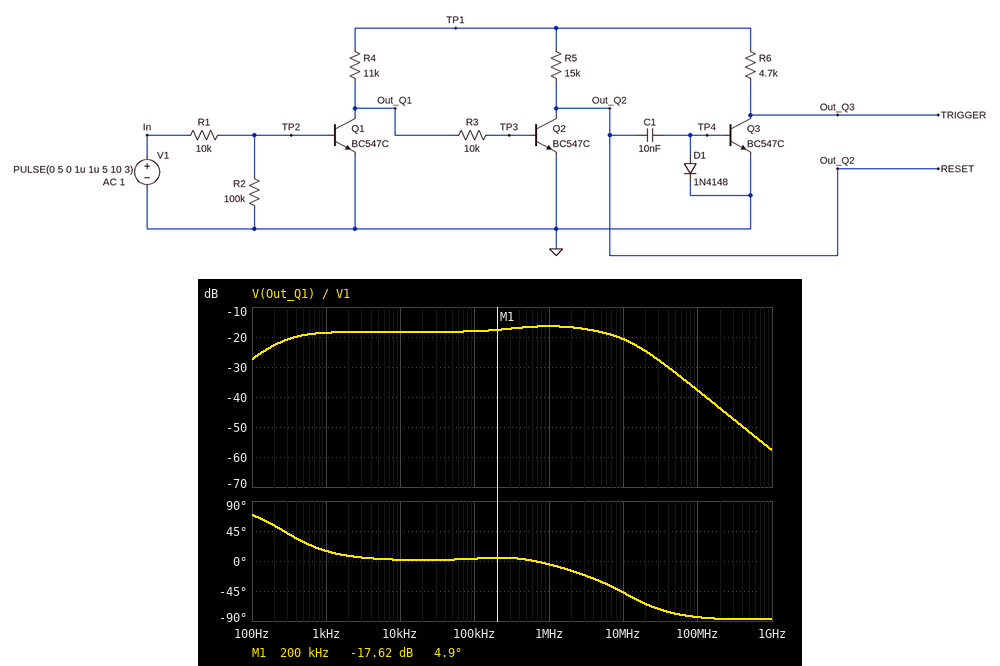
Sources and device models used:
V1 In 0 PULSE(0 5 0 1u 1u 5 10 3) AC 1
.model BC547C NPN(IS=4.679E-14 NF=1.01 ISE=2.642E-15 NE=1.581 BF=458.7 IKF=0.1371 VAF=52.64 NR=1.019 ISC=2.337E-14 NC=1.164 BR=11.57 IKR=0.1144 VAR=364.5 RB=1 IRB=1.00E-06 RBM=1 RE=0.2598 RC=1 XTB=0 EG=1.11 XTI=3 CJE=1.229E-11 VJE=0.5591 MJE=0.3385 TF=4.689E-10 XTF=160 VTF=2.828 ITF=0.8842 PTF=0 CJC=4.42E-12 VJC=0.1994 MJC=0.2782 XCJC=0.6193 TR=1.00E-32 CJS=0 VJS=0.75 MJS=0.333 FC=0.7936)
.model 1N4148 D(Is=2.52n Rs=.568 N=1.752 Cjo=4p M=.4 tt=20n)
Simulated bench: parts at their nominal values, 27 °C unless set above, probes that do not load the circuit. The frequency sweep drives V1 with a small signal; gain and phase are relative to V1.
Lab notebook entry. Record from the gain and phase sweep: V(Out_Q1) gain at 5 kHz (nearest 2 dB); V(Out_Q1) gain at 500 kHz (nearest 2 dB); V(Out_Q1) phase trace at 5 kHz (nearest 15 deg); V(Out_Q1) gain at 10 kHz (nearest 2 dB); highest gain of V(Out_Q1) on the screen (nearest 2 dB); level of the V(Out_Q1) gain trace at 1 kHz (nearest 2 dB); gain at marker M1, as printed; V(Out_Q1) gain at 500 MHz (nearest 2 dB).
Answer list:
-18 dB
-16 dB
0 deg
-18 dB
-16 dB
-18 dB
-17.62 dB
-52 dB
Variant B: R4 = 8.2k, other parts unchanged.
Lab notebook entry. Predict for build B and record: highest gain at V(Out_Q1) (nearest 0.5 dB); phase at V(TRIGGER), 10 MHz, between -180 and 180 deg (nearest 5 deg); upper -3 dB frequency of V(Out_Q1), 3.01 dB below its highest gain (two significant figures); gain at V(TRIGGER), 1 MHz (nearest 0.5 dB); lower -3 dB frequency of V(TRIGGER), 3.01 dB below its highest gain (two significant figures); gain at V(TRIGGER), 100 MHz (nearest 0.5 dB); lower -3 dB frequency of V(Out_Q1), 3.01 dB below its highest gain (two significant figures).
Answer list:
-16.5 dB
-115 deg
6.7 MHz
-18.5 dB
280 Hz
-67.5 dB
440 Hz
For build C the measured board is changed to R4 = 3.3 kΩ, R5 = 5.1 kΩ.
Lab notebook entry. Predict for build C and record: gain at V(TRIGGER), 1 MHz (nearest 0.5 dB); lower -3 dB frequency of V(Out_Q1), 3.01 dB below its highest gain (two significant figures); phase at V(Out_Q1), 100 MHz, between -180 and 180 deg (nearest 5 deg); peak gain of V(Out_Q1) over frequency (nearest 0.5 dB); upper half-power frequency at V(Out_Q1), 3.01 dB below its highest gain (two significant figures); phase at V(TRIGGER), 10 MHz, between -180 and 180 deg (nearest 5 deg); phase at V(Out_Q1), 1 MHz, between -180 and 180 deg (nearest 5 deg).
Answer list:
-19.5 dB
270 Hz
-80 deg
-18.5 dB
5.6 MHz
-100 deg
-10 deg
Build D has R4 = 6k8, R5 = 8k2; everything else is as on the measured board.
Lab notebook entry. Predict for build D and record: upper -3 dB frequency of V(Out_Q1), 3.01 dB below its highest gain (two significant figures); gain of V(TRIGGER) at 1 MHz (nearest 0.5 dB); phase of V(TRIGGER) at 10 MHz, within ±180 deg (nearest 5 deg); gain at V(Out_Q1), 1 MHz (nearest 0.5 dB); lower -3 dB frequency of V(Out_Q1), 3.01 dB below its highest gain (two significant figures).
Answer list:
7.7 MHz
-19.5 dB
-110 deg
-17.5 dB
330 Hz
